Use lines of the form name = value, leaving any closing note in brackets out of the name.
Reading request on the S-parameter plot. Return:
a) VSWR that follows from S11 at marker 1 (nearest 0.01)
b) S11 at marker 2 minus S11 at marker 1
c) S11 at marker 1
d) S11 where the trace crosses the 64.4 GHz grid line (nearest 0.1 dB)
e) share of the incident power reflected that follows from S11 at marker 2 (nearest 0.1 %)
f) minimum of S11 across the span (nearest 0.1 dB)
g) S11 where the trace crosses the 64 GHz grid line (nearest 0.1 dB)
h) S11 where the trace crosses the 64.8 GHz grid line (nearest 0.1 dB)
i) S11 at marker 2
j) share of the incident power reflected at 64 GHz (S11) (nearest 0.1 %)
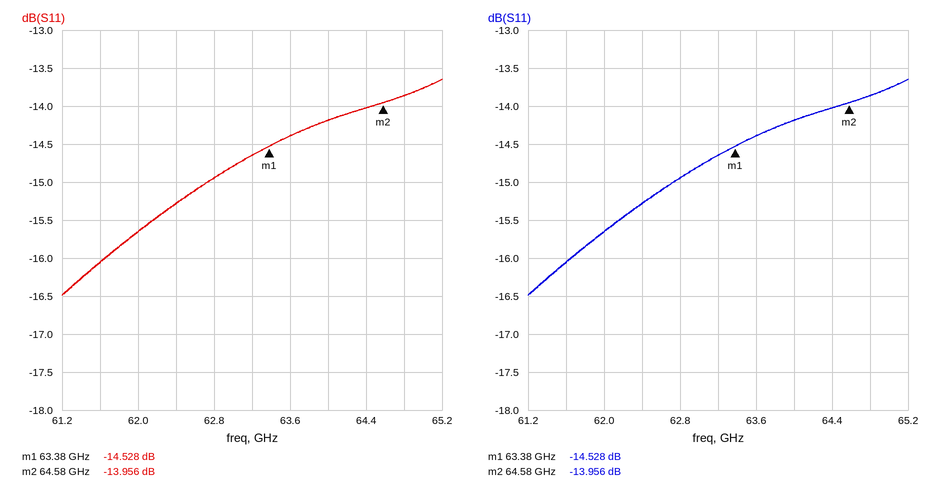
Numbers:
VSWR that follows from S11 at marker 1 = 1.46
S11 at marker 2 minus S11 at marker 1 = 0.572 dB
S11 at marker 1 = -14.528 dB
S11 where the trace crosses the 64.4 GHz grid line = -14.0 dB
share of the incident power reflected that follows from S11 at marker 2 = 4.0 %
minimum of S11 across the span = -16.5 dB
S11 where the trace crosses the 64 GHz grid line = -14.2 dB
S11 where the trace crosses the 64.8 GHz grid line = -13.9 dB
S11 at marker 2 = -13.956 dB
share of the incident power reflected at 64 GHz (S11) = 3.8 %
